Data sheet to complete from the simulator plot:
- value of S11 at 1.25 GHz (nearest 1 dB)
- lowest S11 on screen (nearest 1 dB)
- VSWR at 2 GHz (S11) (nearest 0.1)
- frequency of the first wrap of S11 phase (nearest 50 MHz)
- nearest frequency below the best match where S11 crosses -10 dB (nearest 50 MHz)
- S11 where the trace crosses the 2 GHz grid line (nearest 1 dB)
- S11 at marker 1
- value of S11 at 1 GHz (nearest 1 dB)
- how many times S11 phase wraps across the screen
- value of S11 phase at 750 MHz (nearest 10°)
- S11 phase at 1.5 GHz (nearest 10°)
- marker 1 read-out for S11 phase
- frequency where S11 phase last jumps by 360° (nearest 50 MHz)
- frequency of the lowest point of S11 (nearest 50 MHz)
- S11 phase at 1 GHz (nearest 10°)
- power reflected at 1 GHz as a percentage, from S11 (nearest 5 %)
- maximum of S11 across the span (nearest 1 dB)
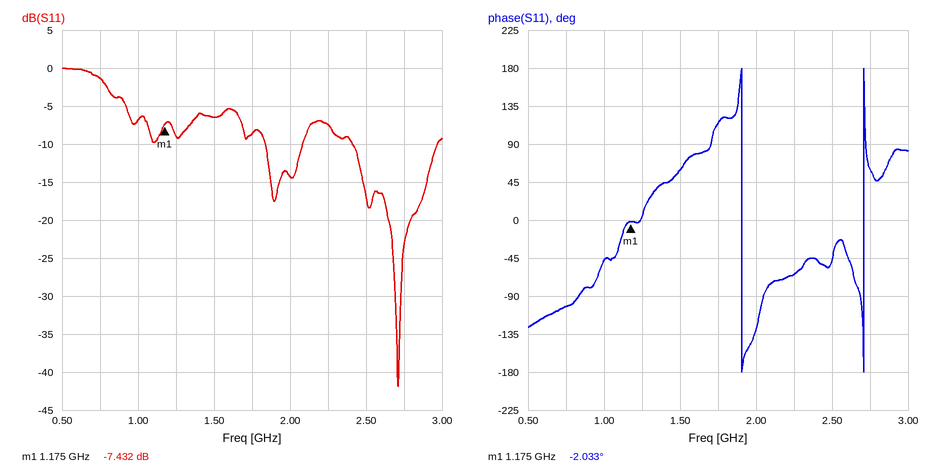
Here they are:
-9 dB
-42 dB
1.5
1.90 GHz
2.40 GHz
-14 dB
-7.432 dB
-7 dB
2
-100°
60°
-2.033°
2.70 GHz
2.70 GHz
-50°
20 %
0 dB
